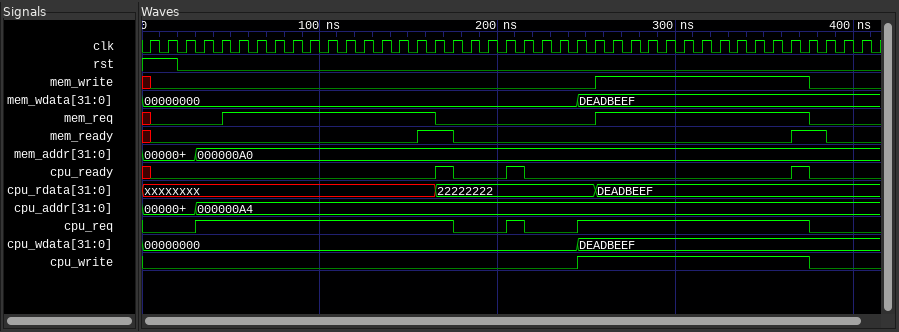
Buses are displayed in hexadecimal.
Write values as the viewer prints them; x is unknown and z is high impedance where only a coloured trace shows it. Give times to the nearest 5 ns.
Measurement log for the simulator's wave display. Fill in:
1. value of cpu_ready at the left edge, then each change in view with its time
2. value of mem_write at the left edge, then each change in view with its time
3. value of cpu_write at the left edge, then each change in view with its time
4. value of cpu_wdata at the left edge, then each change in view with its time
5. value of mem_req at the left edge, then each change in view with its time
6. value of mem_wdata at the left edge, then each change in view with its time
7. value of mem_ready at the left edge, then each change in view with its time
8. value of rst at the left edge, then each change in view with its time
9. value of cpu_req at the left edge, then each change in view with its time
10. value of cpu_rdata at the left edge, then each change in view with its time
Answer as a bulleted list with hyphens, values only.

- x, 0 at 5 ns, 1 at 165 ns, 0 at 175 ns, 1 at 205 ns, 0 at 215 ns, 1 at 365 ns, 0 at 375 ns
- x, 0 at 5 ns, 1 at 255 ns, 0 at 375 ns
- 0, 1 at 245 ns, 0 at 375 ns
- 00000000, DEADBEEF at 245 ns
- x, 0 at 5 ns, 1 at 45 ns, 0 at 165 ns, 1 at 255 ns, 0 at 375 ns
- 00000000, DEADBEEF at 245 ns
- x, 0 at 5 ns, 1 at 155 ns, 0 at 175 ns, 1 at 365 ns, 0 at 385 ns
- 1, 0 at 20 ns
- 0, 1 at 30 ns, 0 at 175 ns, 1 at 205 ns, 0 at 215 ns, 1 at 245 ns, 0 at 375 ns
- xxxxxxxx, 22222222 at 165 ns, DEADBEEF at 255 ns
